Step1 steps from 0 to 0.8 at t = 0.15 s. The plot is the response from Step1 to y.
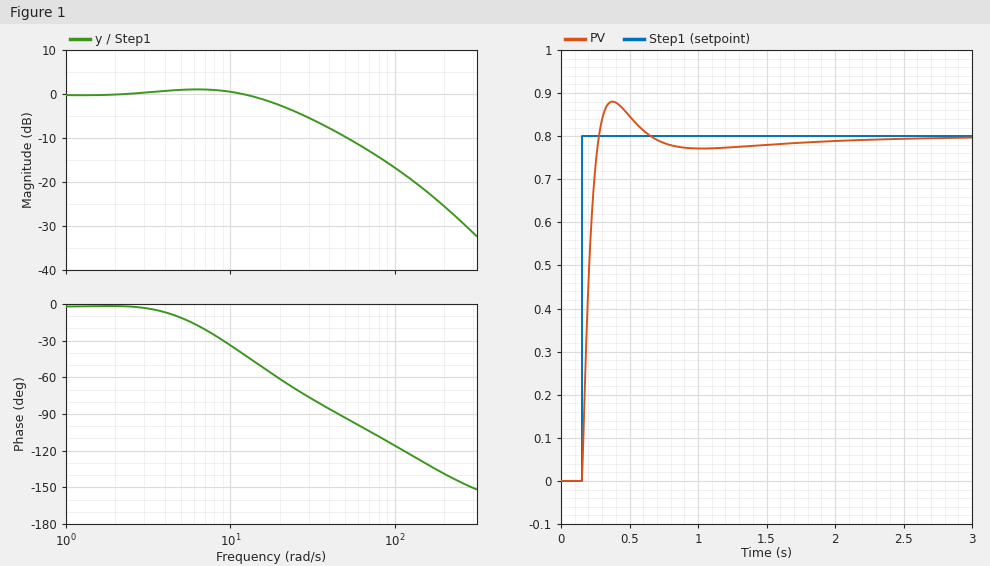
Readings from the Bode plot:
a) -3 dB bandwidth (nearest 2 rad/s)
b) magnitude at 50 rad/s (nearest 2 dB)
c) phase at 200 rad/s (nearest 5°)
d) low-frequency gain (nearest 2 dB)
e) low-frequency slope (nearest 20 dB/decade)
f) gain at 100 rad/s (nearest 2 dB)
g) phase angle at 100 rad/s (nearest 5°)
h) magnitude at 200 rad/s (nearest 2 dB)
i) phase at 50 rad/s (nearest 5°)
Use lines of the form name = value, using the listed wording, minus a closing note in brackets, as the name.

-3 dB bandwidth = 22 rad/s
magnitude at 50 rad/s = -10 dB
phase at 200 rad/s = -140°
low-frequency gain = 0 dB
low-frequency slope = 0 dB/decade
gain at 100 rad/s = -16 dB
phase angle at 100 rad/s = -115°
magnitude at 200 rad/s = -26 dB
phase at 50 rad/s = -95°
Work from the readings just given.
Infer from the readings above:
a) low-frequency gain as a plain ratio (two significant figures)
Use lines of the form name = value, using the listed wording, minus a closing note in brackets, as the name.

low-frequency gain as a plain ratio = 1.0
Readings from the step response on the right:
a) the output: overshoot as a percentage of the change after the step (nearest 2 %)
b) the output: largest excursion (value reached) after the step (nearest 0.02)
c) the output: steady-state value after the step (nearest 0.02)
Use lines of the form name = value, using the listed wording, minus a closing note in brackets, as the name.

the output: overshoot as a percentage of the change after the step = 10 %
the output: largest excursion (value reached) after the step = 0.88
the output: steady-state value after the step = 0.80
